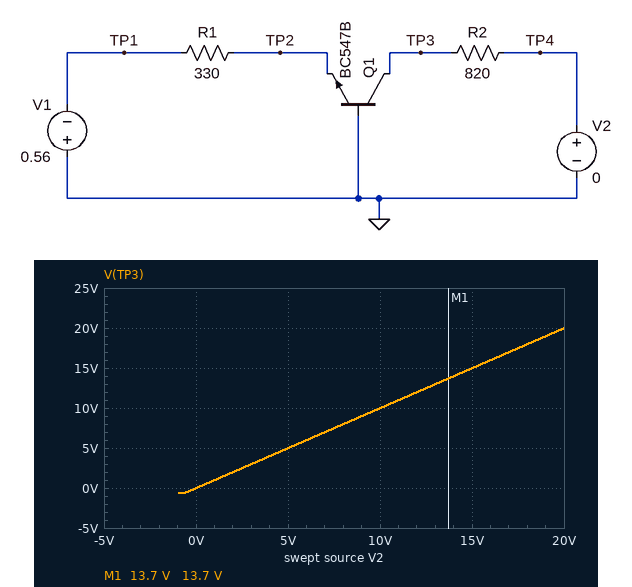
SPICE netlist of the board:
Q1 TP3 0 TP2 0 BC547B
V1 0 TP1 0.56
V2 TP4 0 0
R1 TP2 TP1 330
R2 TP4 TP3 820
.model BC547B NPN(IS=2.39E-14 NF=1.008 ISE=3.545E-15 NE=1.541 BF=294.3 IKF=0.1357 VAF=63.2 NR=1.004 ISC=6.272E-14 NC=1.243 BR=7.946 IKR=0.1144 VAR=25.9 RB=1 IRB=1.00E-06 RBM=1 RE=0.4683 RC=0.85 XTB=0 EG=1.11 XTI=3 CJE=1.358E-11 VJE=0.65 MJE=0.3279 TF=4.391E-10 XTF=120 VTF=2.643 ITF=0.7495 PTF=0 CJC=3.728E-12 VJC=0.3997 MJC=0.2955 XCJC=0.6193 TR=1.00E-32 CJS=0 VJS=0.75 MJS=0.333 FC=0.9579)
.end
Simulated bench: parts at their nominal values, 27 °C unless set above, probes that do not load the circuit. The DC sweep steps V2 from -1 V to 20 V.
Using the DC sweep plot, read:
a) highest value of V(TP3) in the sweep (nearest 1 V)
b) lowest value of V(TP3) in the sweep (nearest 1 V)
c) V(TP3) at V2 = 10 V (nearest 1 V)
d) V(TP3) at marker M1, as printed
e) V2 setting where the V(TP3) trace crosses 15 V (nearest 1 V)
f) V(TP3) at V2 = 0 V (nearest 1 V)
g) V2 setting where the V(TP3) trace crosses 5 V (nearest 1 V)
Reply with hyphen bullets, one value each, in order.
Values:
- 20 V
- -1 V
- 10 V
- 13.7 V
- 15 V
- 0 V
- 5 V
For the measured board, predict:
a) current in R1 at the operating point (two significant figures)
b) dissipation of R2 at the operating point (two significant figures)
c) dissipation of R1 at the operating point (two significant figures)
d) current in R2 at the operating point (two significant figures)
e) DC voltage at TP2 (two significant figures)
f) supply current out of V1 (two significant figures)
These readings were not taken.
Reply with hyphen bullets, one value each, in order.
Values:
- 33 µA
- 880 nW
- 360 nW
- 33 µA
- -550 mV
- 33 µA
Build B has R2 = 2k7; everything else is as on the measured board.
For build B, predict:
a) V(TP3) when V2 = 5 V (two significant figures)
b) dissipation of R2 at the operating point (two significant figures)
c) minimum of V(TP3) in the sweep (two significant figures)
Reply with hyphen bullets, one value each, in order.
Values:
- 4.9 V
- 2.9 µW
- -600 mV
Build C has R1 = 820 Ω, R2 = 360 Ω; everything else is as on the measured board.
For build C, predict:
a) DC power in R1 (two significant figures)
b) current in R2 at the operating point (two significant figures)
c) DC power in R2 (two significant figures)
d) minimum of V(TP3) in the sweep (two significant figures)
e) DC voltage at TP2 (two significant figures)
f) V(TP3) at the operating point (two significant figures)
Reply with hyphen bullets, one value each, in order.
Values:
- 460 nW
- 24 µA
- 200 nW
- -680 mV
- -540 mV
- -8.5 mV
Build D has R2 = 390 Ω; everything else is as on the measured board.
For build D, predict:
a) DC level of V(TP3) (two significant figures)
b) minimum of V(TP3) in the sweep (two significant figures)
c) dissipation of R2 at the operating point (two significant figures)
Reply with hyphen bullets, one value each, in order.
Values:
- -13 mV
- -670 mV
- 420 nW
